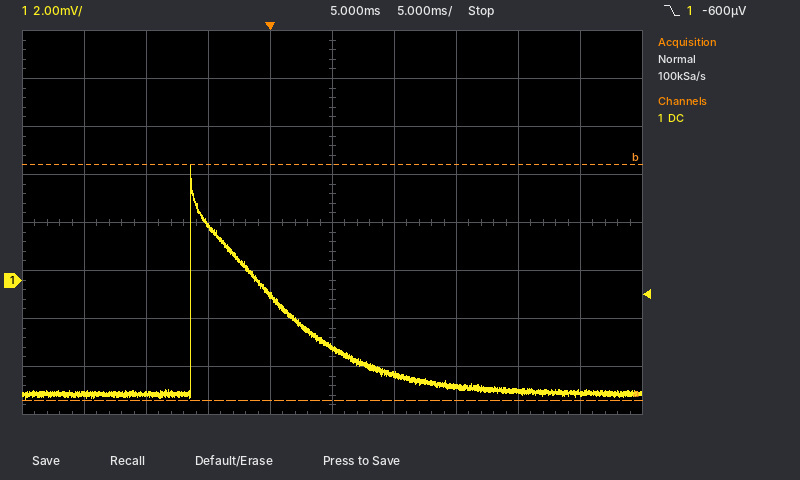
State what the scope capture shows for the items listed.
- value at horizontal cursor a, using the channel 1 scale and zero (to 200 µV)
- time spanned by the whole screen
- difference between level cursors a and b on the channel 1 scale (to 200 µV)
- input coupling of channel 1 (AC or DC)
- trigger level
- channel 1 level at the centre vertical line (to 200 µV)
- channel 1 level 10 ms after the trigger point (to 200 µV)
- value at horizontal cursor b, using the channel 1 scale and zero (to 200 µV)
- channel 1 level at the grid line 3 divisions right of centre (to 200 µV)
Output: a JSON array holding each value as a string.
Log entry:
["-5.0 mV", "50 ms", "9.8 mV", "DC", "-600 µV", "-2.8 mV", "-4.0 mV", "4.8 mV", "-4.6 mV"]
